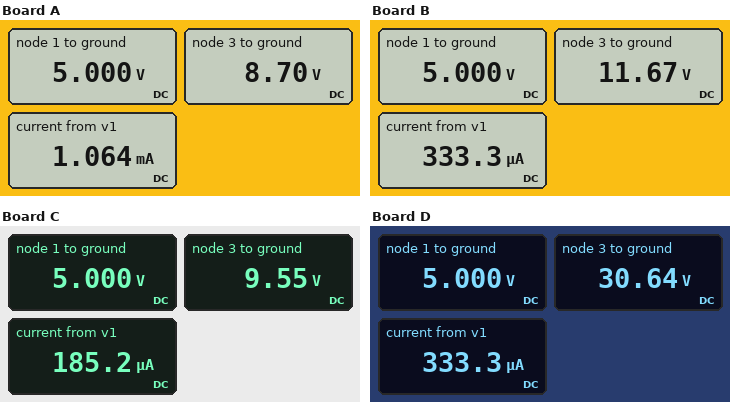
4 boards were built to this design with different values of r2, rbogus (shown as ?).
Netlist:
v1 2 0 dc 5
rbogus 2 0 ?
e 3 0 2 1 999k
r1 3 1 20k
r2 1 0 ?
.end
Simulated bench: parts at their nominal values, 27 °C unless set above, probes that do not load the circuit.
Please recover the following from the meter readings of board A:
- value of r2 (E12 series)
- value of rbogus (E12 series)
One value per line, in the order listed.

27 kΩ
4.7 kΩ
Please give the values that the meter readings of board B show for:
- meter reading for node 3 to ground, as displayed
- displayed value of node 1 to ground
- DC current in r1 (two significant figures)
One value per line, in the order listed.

11.67 V
5.000 V
330 µA
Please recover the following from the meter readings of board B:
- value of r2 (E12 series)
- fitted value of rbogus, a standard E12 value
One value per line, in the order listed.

15 kΩ
15 kΩ
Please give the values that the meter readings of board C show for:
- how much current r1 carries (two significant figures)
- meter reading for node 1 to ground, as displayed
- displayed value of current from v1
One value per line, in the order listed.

230 µA
5.000 V
185.2 µA
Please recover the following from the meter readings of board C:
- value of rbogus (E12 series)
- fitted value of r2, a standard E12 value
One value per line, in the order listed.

27 kΩ
22 kΩ
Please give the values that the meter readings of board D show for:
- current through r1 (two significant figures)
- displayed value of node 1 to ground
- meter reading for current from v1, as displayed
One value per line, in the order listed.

1.3 mA
5.000 V
333.3 µA
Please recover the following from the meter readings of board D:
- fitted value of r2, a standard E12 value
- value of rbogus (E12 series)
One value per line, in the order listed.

3.9 kΩ
15 kΩ
